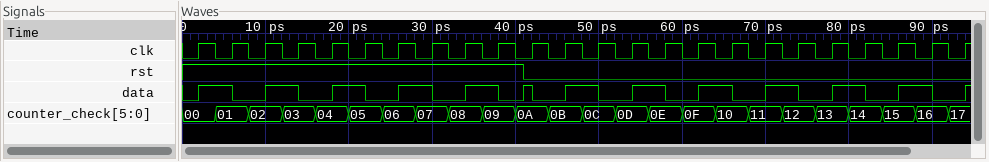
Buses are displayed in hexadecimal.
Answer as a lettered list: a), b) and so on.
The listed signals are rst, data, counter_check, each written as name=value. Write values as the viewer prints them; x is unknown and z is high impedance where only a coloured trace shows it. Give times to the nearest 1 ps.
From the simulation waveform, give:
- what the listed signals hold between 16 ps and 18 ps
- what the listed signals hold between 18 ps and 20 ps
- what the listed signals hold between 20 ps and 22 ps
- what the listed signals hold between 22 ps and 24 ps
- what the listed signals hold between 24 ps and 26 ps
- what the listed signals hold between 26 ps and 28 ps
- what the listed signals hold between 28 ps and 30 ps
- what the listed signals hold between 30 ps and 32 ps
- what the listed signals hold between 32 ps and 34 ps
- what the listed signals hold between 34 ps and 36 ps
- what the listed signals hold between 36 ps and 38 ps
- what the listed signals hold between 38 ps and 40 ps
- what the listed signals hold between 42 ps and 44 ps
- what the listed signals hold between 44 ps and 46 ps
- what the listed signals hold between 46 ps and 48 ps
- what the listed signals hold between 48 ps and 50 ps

a) rst=1, data=0, counter_check=04
b) rst=1, data=1, counter_check=04
c) rst=1, data=1, counter_check=05
d) rst=1, data=0, counter_check=05
e) rst=1, data=0, counter_check=06
f) rst=1, data=1, counter_check=06
g) rst=1, data=1, counter_check=07
h) rst=1, data=0, counter_check=07
i) rst=1, data=0, counter_check=08
j) rst=1, data=1, counter_check=08
k) rst=1, data=1, counter_check=09
l) rst=1, data=0, counter_check=09
m) rst=0, data=0, counter_check=0A
n) rst=0, data=0, counter_check=0B
o) rst=0, data=1, counter_check=0B
p) rst=0, data=1, counter_check=0C
